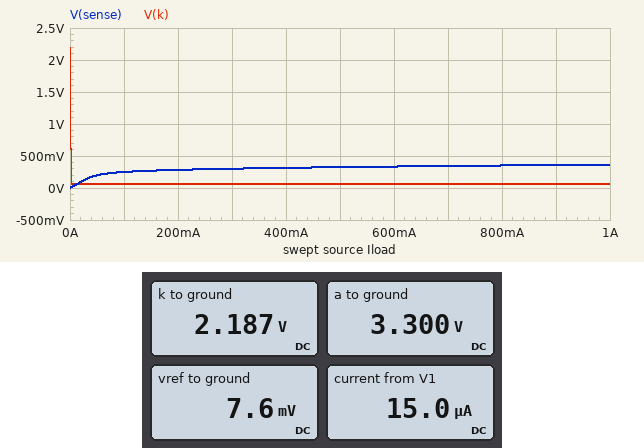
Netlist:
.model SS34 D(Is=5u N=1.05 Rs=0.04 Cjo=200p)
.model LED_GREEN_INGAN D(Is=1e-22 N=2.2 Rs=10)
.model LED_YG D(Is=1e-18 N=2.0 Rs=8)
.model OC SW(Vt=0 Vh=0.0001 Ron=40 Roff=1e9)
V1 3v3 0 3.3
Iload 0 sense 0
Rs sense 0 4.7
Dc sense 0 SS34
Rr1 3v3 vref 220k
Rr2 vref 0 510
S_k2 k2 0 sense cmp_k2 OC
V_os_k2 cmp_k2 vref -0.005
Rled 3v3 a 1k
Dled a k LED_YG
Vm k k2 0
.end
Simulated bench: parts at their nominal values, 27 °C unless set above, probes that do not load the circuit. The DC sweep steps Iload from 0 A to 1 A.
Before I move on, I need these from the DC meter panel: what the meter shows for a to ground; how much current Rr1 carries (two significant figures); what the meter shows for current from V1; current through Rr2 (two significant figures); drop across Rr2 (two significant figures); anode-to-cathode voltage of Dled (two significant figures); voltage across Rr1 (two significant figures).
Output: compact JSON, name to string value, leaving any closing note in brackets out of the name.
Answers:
{"what the meter shows for a to ground": "3.300 V", "how much current Rr1 carries": "15 µA", "what the meter shows for current from V1": "15.0 µA", "current through Rr2": "15 µA", "drop across Rr2": "7.6 mV", "anode-to-cathode voltage of Dled": "1.1 V", "voltage across Rr1": "3.3 V"}
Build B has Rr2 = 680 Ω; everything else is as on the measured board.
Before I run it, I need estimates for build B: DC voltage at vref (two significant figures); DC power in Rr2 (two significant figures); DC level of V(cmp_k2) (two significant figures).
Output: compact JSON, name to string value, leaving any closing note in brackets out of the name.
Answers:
{"DC voltage at vref": "10 mV", "DC power in Rr2": "150 nW", "DC level of V(cmp_k2)": "5.2 mV"}
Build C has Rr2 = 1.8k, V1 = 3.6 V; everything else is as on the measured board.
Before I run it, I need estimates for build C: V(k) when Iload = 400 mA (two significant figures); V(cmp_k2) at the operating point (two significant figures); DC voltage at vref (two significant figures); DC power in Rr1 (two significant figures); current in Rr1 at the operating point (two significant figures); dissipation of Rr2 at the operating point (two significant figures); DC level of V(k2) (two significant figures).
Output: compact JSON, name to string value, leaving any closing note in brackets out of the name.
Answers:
{"V(k) when Iload = 400 mA": "68 mV", "V(cmp_k2) at the operating point": "24 mV", "DC voltage at vref": "29 mV", "DC power in Rr1": "58 µW", "current in Rr1 at the operating point": "16 µA", "dissipation of Rr2 at the operating point": "470 nW", "DC level of V(k2)": "2.5 V"}
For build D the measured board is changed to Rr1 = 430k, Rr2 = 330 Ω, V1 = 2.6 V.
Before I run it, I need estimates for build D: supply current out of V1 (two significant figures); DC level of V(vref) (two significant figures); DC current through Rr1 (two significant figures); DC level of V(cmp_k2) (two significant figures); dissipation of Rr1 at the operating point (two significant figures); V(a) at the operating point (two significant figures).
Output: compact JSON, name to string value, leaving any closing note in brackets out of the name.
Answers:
{"supply current out of V1": "790 µA", "DC level of V(vref)": "2.0 mV", "DC current through Rr1": "6.0 µA", "DC level of V(cmp_k2)": "-3.0 mV", "dissipation of Rr1 at the operating point": "16 µW", "V(a) at the operating point": "1.8 V"}
